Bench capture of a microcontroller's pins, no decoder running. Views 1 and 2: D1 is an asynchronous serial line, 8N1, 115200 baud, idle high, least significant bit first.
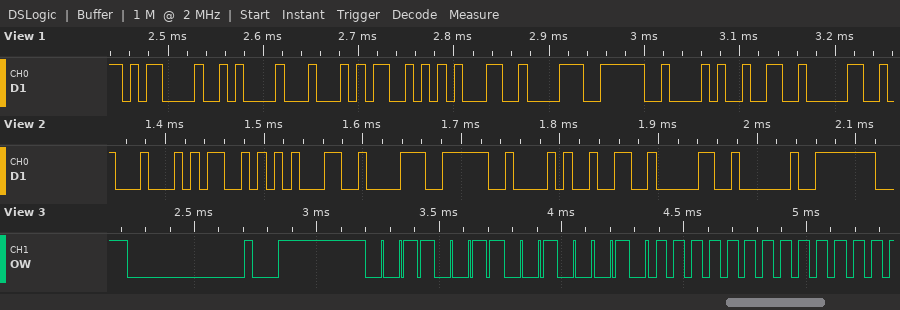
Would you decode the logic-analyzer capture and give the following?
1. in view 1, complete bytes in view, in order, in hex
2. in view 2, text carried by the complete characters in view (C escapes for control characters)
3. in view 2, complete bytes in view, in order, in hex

0x0D 0x0A 0x44 0x53 0x31 0x38 0x42 0x32 0x30
"DS18B20 "
44 53 31 38 42 32 30 20
